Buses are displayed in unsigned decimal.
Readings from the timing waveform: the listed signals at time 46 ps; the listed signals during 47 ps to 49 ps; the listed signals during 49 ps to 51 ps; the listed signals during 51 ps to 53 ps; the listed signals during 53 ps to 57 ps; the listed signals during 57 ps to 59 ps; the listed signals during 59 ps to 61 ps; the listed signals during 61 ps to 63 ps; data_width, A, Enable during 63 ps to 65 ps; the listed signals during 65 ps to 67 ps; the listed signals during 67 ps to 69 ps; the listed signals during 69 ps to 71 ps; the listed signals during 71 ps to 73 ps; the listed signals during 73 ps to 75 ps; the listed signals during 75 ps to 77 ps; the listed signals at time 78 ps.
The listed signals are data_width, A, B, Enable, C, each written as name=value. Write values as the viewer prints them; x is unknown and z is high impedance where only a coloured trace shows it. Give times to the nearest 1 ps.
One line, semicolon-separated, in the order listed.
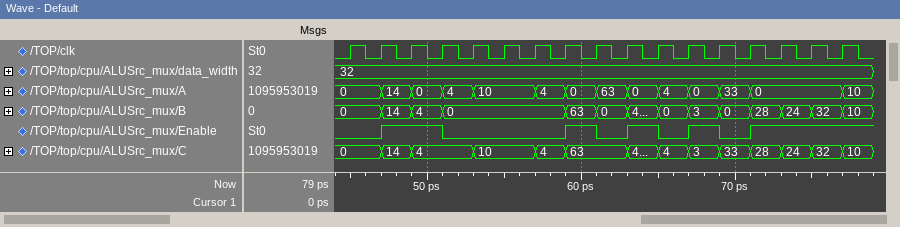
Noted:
data_width=32, A=0, B=0, Enable=0, C=0; data_width=32, A=14, B=14, Enable=1, C=14; data_width=32, A=0, B=4, Enable=1, C=4; data_width=32, A=4, B=0, Enable=0, C=4; data_width=32, A=10, B=0, Enable=0, C=10; data_width=32, A=4, B=0, Enable=0, C=4; data_width=32, A=0, B=63, Enable=1, C=63; data_width=32, A=63, B=0, Enable=0, C=63; data_width=32, A=0, Enable=1; data_width=32, A=4, B=0, Enable=0, C=4; data_width=32, A=0, B=3, Enable=1, C=3; data_width=32, A=33, B=0, Enable=0, C=33; data_width=32, A=0, B=28, Enable=1, C=28; data_width=32, A=0, B=24, Enable=1, C=24; data_width=32, A=0, B=32, Enable=1, C=32; data_width=32, A=10, B=10, Enable=1, C=10
